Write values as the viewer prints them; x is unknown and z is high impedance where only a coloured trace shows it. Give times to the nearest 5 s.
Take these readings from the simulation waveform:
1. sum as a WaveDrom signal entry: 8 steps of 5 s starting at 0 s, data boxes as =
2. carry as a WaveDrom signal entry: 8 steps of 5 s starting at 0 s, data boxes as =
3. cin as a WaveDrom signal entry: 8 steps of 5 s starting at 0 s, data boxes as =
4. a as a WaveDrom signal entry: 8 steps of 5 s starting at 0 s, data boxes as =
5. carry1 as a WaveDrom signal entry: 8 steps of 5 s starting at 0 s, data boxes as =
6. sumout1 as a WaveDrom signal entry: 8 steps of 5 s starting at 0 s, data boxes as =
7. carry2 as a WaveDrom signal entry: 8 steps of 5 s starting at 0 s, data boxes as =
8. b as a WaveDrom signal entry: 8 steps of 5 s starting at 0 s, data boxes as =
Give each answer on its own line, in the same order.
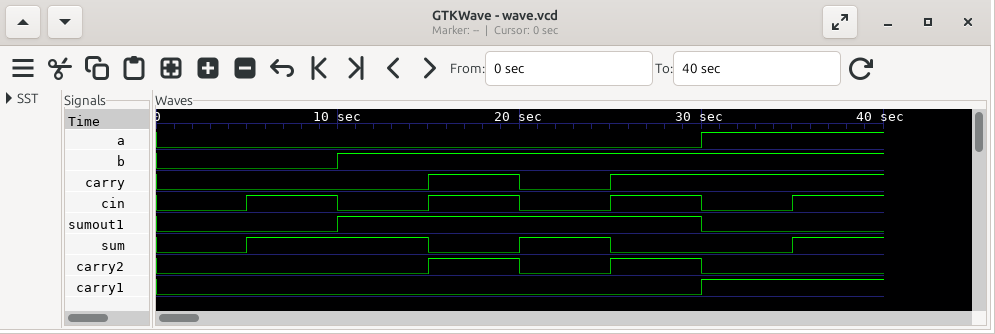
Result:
{name: 'sum', wave: '01.010.1'}
{name: 'carry', wave: '0..101..'}
{name: 'cin', wave: '01010101'}
{name: 'a', wave: '0.....1.'}
{name: 'carry1', wave: '0.....1.'}
{name: 'sumout1', wave: '0.1...0.'}
{name: 'carry2', wave: '0..1010.'}
{name: 'b', wave: '0.1.....'}
